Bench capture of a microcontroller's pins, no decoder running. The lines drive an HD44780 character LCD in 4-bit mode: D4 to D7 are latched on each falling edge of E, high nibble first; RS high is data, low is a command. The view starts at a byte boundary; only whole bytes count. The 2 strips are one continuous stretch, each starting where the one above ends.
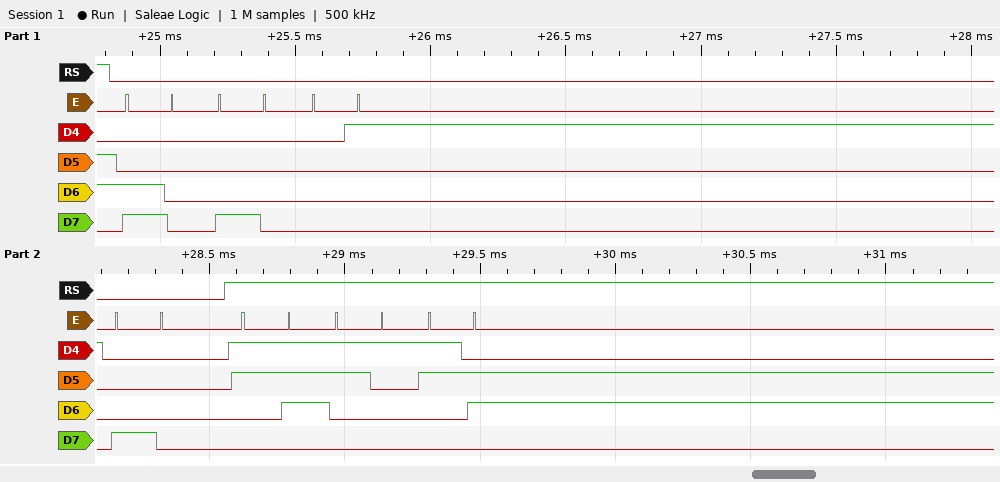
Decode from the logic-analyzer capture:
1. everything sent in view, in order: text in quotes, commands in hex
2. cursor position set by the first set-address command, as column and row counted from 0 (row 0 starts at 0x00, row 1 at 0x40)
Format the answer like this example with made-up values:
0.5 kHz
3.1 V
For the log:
0xC0 0x80 0x01 0x80 "716"
column 0, row 1
